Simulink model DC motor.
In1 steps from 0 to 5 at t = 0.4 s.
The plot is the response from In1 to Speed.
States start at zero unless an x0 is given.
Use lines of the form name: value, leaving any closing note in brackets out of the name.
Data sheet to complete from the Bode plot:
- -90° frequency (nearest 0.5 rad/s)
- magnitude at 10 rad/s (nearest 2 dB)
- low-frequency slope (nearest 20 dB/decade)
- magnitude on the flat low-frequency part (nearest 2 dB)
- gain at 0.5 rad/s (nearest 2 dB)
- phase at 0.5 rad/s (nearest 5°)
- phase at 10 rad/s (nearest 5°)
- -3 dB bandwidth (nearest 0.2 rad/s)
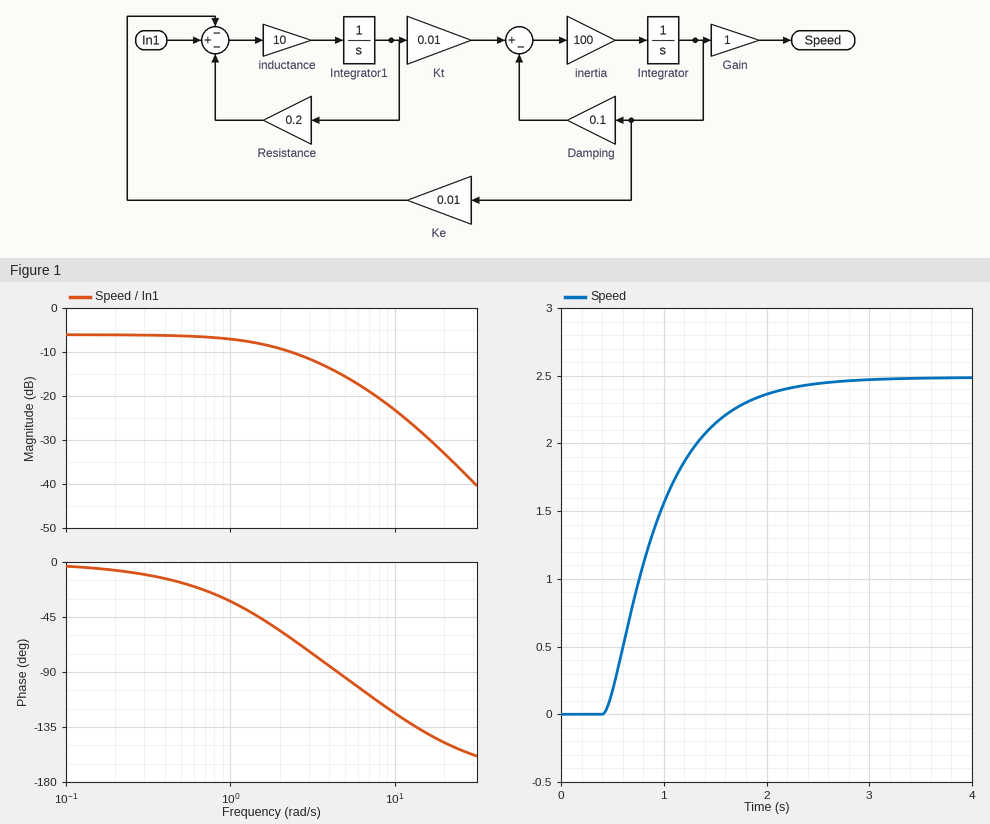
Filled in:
-90° frequency: 4.5 rad/s
magnitude at 10 rad/s: -24 dB
low-frequency slope: 0 dB/decade
magnitude on the flat low-frequency part: -6 dB
gain at 0.5 rad/s: -6 dB
phase at 0.5 rad/s: -15°
phase at 10 rad/s: -125°
-3 dB bandwidth: 2.0 rad/s
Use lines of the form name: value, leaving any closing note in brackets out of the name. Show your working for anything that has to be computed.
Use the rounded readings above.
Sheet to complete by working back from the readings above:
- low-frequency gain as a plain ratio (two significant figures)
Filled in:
low-frequency gain as a plain ratio: 10^(-6 / 20) = 0.50
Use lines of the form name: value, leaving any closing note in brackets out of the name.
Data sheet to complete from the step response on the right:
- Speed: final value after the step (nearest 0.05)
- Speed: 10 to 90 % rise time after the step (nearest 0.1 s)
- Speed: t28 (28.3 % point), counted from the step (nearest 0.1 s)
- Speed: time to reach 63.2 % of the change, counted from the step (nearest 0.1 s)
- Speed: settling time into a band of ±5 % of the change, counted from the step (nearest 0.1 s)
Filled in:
Speed: final value after the step: 2.50
Speed: 10 to 90 % rise time after the step: 1.1 s
Speed: t28 (28.3 % point), counted from the step: 0.3 s
Speed: time to reach 63.2 % of the change, counted from the step: 0.6 s
Speed: settling time into a band of ±5 % of the change, counted from the step: 1.6 s
